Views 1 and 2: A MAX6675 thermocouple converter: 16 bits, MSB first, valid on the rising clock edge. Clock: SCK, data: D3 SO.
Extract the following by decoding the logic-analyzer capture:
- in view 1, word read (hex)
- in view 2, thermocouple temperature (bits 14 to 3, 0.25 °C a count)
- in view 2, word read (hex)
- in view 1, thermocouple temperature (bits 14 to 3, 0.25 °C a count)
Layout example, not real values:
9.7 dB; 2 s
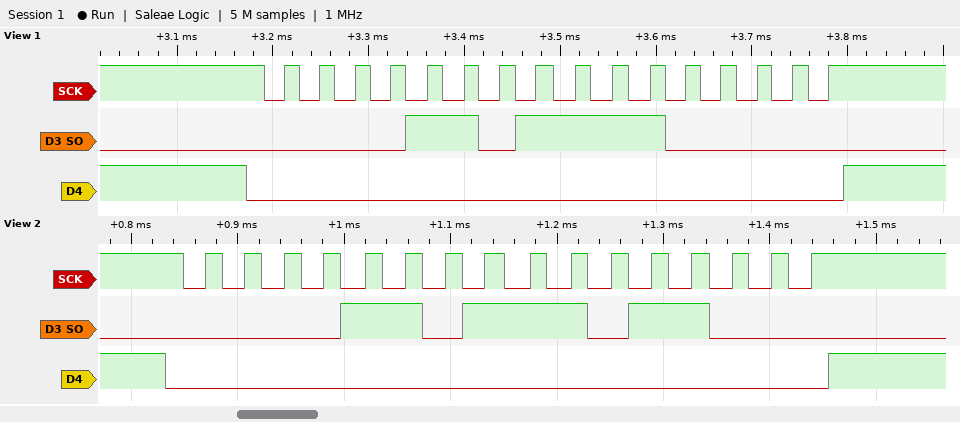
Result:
0x0DE0; 110.75 °C; 0x0DD8; 111.00 °C
